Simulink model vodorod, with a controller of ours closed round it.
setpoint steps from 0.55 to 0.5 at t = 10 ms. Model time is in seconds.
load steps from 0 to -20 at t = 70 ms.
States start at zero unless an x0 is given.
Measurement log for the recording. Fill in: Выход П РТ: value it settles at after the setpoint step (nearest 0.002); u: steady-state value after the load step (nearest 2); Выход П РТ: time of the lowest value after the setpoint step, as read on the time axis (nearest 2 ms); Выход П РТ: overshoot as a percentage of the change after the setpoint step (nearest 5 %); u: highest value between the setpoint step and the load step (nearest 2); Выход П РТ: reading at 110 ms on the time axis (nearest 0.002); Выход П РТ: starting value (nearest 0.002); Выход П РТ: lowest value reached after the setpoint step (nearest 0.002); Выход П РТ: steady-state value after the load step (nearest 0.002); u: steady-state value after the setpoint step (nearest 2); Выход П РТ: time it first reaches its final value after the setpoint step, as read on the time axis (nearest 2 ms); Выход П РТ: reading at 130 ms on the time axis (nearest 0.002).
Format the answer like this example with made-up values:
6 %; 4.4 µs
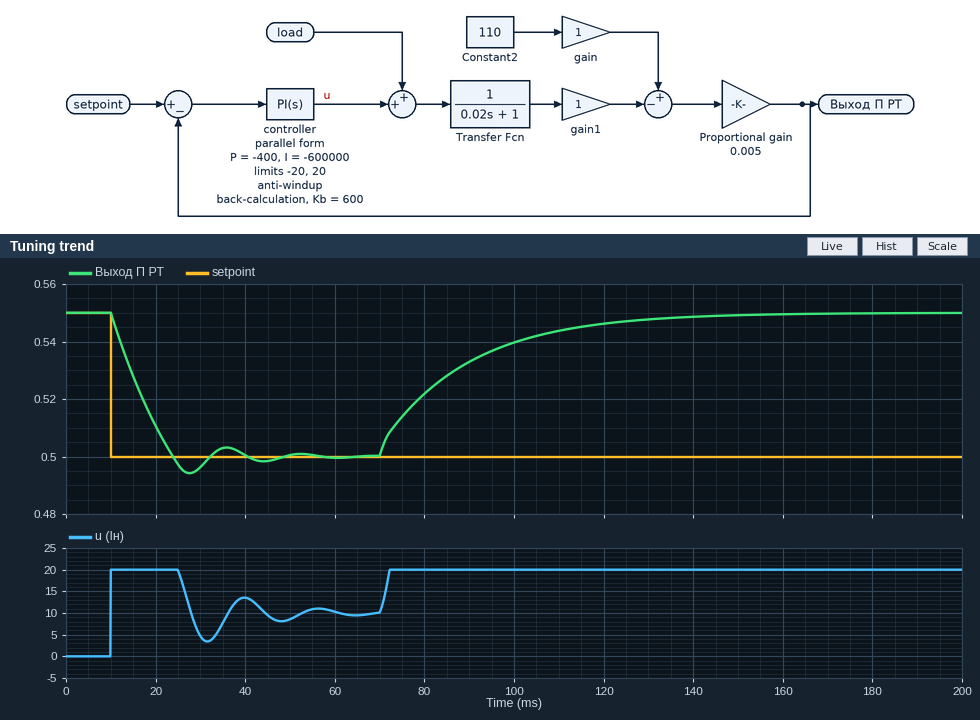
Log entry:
0.500; 20; 28 ms; 10 %; 20; 0.544; 0.550; 0.494; 0.550; 10; 24 ms; 0.548
